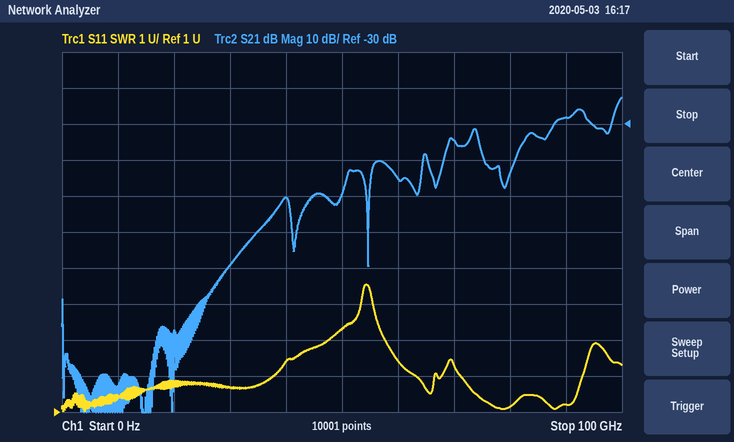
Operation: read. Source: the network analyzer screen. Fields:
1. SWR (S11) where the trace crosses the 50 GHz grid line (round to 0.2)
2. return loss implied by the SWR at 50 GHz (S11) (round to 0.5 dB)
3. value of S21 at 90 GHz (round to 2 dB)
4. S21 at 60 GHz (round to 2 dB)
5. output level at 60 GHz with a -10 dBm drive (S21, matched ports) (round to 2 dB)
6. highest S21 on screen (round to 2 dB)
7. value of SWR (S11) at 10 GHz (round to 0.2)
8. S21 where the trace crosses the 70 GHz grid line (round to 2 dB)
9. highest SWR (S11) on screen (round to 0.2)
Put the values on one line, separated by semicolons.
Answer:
3.4; 5.5 dB; -28 dB; -46 dB; -56 dBm; -22 dB; 1.4; -34 dB; 4.6
